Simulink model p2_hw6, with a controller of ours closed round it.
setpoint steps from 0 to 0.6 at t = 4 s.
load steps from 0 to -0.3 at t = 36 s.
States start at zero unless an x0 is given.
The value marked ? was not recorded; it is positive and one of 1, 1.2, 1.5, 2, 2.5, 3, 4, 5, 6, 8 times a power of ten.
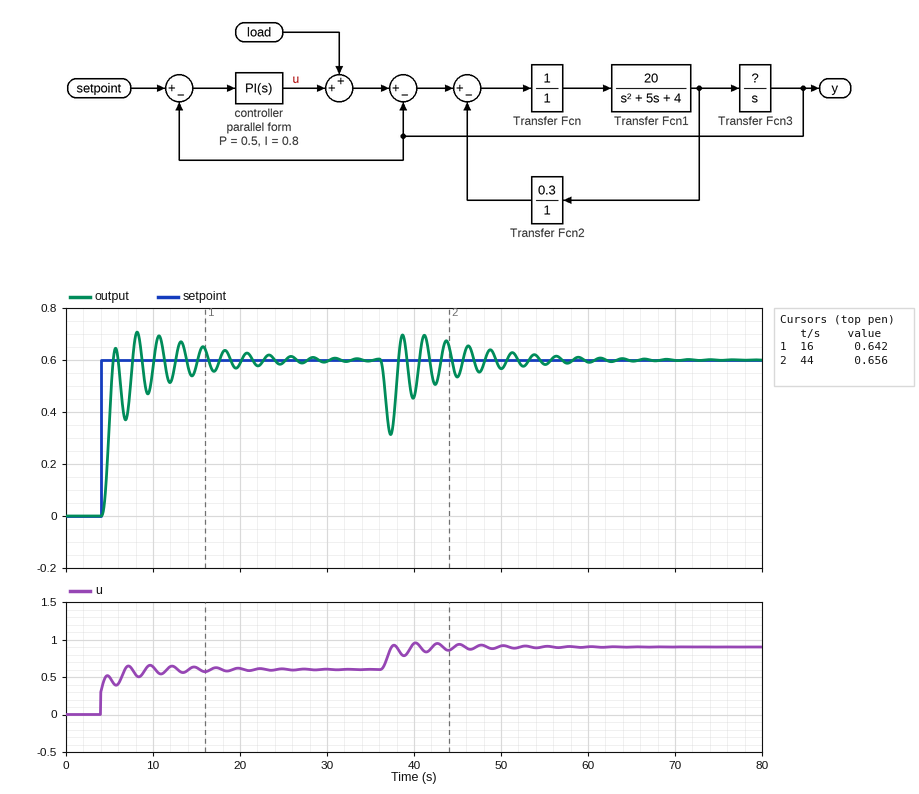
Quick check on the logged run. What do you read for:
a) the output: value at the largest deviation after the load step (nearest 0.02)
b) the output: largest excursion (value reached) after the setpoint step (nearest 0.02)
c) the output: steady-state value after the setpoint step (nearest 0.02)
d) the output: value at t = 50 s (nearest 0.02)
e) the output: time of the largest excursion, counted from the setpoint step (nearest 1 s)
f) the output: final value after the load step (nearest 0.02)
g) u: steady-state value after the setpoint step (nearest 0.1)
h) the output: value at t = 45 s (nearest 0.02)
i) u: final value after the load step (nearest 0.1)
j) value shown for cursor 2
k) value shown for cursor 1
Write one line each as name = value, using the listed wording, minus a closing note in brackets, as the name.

the output: value at the largest deviation after the load step = 0.32
the output: largest excursion (value reached) after the setpoint step = 0.70
the output: steady-state value after the setpoint step = 0.60
the output: value at t = 50 s = 0.56
the output: time of the largest excursion, counted from the setpoint step = 4 s
the output: final value after the load step = 0.60
u: steady-state value after the setpoint step = 0.6
the output: value at t = 45 s = 0.54
u: final value after the load step = 0.9
value shown for cursor 2 = 0.656
value shown for cursor 1 = 0.642
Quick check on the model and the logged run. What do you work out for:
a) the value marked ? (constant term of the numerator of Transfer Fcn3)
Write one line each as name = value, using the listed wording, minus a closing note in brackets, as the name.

the value marked ? = 1
